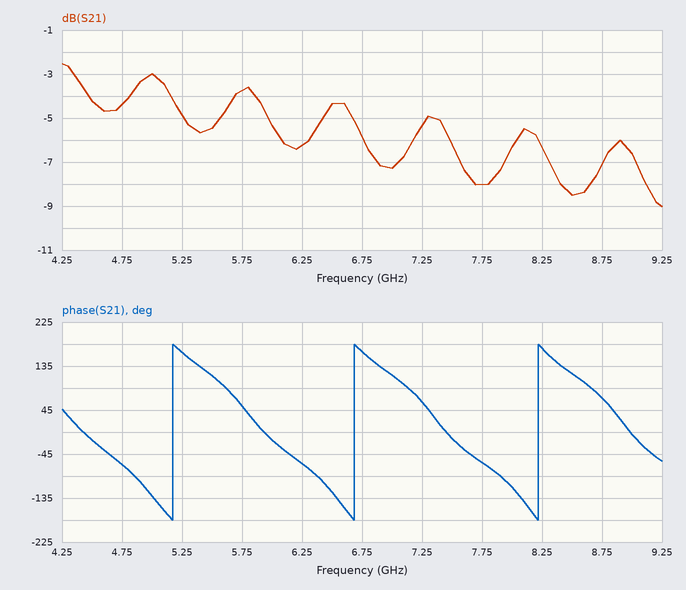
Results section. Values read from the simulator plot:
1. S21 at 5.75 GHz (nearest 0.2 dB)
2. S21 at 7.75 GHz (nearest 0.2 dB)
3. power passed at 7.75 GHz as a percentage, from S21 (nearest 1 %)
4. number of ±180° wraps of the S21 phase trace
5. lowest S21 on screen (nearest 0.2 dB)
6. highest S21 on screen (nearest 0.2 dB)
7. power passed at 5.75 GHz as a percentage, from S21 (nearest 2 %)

-3.8 dB
-8.0 dB
16 %
3
-9.0 dB
-2.6 dB
42 %
